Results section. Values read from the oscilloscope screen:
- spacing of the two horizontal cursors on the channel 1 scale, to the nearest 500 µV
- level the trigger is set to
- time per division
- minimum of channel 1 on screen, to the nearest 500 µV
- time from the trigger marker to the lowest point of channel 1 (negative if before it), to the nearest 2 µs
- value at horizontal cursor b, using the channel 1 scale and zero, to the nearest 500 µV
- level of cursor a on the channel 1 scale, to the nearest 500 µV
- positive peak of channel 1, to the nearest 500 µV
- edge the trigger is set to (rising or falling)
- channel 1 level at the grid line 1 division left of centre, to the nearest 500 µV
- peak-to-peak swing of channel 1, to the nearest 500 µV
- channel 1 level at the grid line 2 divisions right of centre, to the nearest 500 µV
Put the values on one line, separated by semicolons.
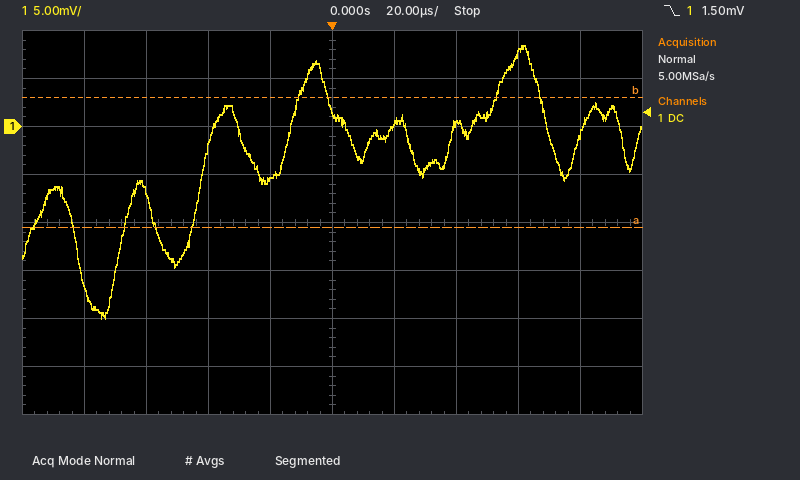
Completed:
13.5 mV; 1.50 mV; 20 µs; -20.0 mV; -74 µs; 3.0 mV; -10.5 mV; 8.5 mV; falling; -5.5 mV; 28.5 mV; 0.0 mV
